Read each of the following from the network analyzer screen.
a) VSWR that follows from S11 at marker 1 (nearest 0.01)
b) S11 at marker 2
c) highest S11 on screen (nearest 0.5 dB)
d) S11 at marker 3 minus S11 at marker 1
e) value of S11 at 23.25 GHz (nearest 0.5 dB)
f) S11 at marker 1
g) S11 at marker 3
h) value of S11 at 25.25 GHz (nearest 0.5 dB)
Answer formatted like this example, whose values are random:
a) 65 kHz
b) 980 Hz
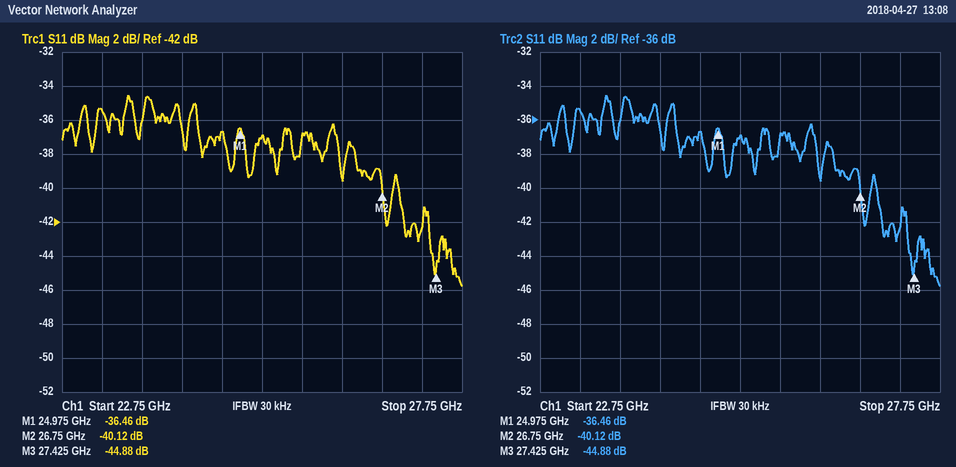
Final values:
a) 1.03
b) -40.12 dB
c) -34.5 dB
d) -8.42 dB
e) -35.5 dB
f) -36.46 dB
g) -44.88 dB
h) -37.0 dB
